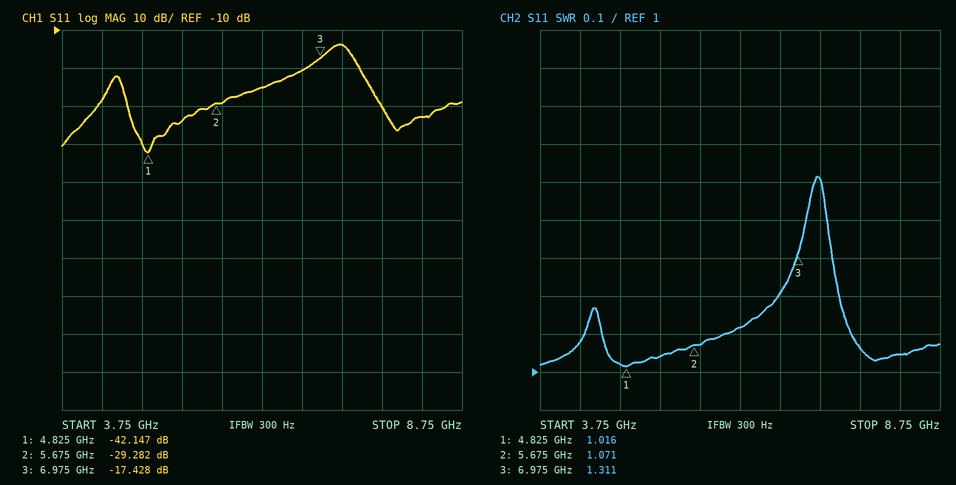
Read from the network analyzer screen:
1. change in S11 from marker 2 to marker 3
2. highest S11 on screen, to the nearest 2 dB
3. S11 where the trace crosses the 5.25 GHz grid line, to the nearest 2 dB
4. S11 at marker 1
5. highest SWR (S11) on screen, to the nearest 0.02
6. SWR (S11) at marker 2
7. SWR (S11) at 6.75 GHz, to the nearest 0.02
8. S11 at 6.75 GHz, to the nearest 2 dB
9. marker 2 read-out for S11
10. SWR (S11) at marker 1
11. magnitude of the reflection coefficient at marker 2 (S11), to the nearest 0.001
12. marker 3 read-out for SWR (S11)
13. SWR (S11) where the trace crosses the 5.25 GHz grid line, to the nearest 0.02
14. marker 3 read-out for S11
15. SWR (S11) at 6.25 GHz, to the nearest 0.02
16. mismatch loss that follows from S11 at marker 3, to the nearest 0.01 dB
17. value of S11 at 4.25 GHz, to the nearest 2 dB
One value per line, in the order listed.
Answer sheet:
11.854 dB
-14 dB
-34 dB
-42.147 dB
1.52
1.071
1.20
-20 dB
-29.282 dB
1.016
0.034
1.311
1.04
-17.428 dB
1.12
0.08 dB
-28 dB
